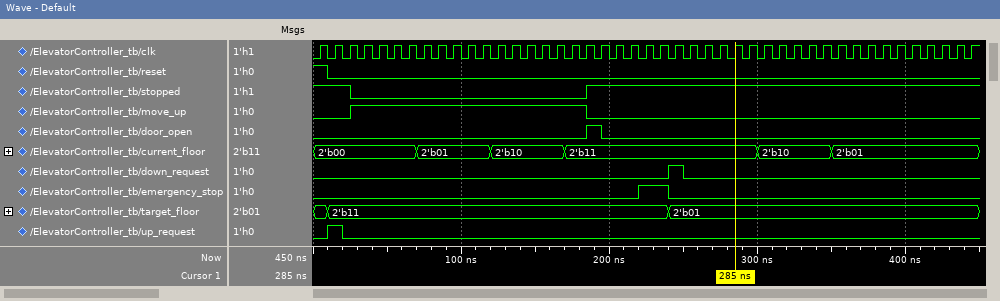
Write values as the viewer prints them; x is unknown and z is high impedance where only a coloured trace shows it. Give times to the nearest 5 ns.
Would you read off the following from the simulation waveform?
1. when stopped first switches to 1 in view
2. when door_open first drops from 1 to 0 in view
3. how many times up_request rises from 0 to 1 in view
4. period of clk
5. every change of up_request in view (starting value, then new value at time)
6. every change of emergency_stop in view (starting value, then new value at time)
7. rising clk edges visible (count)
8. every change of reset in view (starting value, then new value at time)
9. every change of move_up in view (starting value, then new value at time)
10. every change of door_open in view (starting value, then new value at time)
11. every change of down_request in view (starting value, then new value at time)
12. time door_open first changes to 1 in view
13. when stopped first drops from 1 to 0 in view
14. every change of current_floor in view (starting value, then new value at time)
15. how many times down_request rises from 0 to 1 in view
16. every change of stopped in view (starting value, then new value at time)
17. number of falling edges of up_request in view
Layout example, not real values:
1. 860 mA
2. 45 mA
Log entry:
1. 185 ns
2. 195 ns
3. 1
4. 10 ns
5. 0, 1 at 10 ns, 0 at 20 ns
6. 0, 1 at 220 ns, 0 at 240 ns
7. 45
8. 1, 0 at 10 ns
9. 0, 1 at 25 ns, 0 at 185 ns
10. 0, 1 at 185 ns, 0 at 195 ns
11. 0, 1 at 240 ns, 0 at 250 ns
12. 185 ns
13. 25 ns
14. 2'b00, 2'b01 at 70 ns, 2'b10 at 120 ns, 2'b11 at 170 ns, 2'b10 at 300 ns, 2'b01 at 350 ns
15. 1
16. 1, 0 at 25 ns, 1 at 185 ns
17. 1
